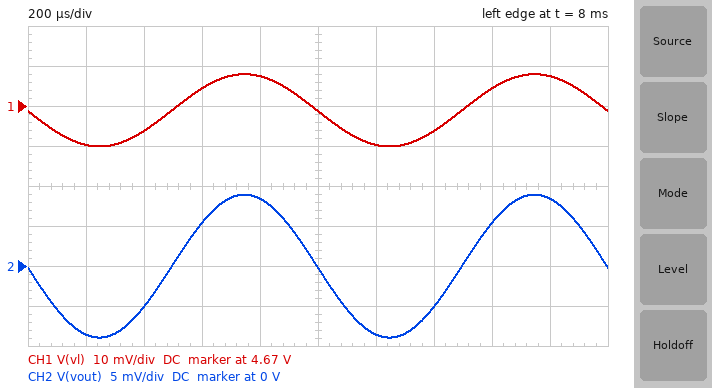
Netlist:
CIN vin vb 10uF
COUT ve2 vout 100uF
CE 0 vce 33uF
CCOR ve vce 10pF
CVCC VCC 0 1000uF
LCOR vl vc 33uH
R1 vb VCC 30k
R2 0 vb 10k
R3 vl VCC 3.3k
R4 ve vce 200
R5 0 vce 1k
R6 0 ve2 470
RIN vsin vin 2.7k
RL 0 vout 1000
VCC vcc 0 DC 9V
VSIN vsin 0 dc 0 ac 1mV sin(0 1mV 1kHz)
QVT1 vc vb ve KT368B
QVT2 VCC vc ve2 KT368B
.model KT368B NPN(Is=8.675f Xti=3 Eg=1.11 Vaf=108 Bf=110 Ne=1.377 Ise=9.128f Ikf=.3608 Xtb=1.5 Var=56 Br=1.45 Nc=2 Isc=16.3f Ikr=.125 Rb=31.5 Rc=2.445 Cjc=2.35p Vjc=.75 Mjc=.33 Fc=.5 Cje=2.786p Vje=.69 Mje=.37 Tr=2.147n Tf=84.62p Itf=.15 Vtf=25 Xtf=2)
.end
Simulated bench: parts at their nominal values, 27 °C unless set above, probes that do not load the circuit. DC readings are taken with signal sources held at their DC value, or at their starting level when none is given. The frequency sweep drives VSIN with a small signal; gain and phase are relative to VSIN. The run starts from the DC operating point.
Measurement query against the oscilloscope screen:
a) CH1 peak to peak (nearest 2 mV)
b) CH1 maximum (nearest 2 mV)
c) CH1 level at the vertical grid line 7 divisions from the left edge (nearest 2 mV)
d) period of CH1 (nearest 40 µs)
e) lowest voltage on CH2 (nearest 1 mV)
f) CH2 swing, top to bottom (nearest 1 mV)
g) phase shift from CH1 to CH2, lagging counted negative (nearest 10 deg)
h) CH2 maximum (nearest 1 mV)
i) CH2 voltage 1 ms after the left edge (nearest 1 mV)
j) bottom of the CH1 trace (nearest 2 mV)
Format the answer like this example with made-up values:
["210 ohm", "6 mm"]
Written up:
["18 mV", "4.678 V", "4.664 V", "1.00 ms", "-9 mV", "18 mV", "0 deg", "9 mV", "0 V", "4.660 V"]
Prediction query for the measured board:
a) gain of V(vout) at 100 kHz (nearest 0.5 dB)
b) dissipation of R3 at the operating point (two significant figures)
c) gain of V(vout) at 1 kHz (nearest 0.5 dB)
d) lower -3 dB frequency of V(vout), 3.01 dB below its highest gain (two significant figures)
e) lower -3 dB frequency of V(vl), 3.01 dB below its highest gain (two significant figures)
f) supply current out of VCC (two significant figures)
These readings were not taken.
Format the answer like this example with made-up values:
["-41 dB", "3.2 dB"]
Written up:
["19.0 dB", "5.7 mW", "19.0 dB", "24 Hz", "24 Hz", "9.9 mA"]
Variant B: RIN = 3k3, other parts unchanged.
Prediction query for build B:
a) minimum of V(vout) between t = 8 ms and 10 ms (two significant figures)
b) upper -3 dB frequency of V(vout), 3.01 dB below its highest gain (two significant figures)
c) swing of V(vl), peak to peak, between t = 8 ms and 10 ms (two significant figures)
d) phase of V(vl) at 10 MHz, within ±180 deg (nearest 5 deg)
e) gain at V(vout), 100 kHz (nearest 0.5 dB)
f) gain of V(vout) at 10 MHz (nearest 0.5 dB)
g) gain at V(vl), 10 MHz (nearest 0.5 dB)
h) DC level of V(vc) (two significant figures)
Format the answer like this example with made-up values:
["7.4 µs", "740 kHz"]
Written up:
["-8.3 mV", "3.7 MHz", "17 mV", "70 deg", "18.5 dB", "9.0 dB", "7.5 dB", "4.7 V"]
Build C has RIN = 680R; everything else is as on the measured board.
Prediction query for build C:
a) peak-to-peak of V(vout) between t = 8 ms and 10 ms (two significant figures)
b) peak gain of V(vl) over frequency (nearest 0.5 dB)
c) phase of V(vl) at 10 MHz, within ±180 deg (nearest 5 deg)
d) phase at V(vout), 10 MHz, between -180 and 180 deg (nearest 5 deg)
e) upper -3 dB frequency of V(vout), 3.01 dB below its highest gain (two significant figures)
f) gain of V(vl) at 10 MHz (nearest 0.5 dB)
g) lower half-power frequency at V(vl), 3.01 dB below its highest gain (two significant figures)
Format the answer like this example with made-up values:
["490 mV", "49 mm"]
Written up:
["24 mV", "21.5 dB", "95 deg", "130 deg", "13 MHz", "18.5 dB", "26 Hz"]
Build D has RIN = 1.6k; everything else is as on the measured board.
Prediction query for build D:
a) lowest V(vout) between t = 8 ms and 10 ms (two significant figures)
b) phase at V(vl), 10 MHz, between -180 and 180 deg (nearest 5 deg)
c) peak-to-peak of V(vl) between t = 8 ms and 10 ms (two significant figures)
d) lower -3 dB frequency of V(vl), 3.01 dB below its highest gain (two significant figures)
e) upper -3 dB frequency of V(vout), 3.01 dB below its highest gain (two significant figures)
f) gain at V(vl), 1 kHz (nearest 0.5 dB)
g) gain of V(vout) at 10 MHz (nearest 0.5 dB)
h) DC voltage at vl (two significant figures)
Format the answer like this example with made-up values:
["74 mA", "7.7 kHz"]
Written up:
["-10 mV", "80 deg", "21 mV", "25 Hz", "6.5 MHz", "20.5 dB", "14.5 dB", "4.7 V"]
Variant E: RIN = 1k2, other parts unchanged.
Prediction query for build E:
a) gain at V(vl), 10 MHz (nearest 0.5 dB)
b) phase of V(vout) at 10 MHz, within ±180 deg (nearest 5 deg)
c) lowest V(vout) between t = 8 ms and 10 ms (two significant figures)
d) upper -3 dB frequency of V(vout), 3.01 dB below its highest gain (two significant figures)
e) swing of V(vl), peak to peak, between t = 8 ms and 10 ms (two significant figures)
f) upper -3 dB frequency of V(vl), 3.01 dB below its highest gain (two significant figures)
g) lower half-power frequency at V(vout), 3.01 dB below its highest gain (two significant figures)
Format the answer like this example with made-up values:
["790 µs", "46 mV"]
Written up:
["15.0 dB", "115 deg", "-11 mV", "8.2 MHz", "22 mV", "7.0 MHz", "25 Hz"]
